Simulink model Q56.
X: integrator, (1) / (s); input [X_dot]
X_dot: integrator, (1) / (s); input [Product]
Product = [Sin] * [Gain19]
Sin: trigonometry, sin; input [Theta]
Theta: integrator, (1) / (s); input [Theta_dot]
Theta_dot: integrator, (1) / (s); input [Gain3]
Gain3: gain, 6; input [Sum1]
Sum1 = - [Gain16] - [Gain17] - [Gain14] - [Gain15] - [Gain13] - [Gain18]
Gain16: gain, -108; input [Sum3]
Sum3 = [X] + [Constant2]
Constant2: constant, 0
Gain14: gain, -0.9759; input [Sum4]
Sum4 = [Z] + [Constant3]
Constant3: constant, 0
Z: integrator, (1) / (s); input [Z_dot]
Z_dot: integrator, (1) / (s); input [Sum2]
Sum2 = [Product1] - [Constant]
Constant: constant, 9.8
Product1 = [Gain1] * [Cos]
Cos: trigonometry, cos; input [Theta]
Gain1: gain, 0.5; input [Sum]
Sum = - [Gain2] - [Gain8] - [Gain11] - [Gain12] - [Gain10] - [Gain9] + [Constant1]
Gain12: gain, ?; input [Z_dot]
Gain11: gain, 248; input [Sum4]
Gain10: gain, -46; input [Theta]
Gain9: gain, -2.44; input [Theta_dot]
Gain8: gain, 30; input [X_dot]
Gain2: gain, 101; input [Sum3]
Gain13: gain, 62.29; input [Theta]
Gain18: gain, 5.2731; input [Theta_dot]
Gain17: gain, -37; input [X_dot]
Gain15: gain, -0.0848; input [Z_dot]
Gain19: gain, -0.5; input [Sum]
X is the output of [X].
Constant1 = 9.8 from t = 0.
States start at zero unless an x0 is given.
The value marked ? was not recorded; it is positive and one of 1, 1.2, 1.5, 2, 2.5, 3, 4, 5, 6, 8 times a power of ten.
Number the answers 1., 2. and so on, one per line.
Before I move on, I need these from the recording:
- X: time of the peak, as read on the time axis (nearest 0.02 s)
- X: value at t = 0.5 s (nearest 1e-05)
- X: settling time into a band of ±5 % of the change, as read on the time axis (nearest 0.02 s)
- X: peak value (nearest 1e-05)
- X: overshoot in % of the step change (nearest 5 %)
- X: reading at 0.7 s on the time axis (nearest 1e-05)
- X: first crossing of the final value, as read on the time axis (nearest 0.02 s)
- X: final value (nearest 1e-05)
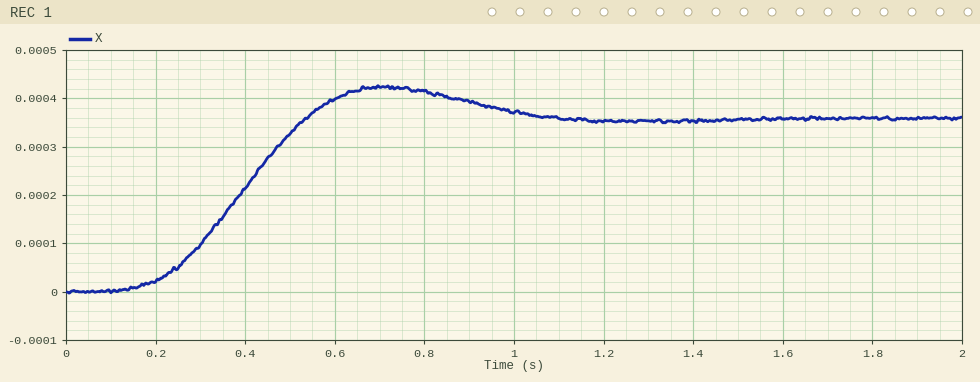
1. 0.72 s
2. 0.00033
3. 0.98 s
4. 0.00042
5. 20 %
6. 0.00042
7. 0.54 s
8. 0.00036
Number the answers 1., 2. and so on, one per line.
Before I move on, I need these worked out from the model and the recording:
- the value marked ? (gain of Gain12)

1. 20
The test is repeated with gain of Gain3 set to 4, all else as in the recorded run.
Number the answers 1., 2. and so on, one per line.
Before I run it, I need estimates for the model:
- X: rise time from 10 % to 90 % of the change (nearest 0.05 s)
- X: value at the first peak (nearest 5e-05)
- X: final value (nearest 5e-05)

1. 0.25 s
2. 0.00045
3. 0.00035
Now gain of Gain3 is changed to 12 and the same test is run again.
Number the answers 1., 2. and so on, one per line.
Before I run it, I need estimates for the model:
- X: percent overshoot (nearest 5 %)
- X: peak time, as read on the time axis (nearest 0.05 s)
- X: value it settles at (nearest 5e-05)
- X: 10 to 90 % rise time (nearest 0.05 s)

1. 15 %
2. 0.75 s
3. 0.00035
4. 0.30 s
